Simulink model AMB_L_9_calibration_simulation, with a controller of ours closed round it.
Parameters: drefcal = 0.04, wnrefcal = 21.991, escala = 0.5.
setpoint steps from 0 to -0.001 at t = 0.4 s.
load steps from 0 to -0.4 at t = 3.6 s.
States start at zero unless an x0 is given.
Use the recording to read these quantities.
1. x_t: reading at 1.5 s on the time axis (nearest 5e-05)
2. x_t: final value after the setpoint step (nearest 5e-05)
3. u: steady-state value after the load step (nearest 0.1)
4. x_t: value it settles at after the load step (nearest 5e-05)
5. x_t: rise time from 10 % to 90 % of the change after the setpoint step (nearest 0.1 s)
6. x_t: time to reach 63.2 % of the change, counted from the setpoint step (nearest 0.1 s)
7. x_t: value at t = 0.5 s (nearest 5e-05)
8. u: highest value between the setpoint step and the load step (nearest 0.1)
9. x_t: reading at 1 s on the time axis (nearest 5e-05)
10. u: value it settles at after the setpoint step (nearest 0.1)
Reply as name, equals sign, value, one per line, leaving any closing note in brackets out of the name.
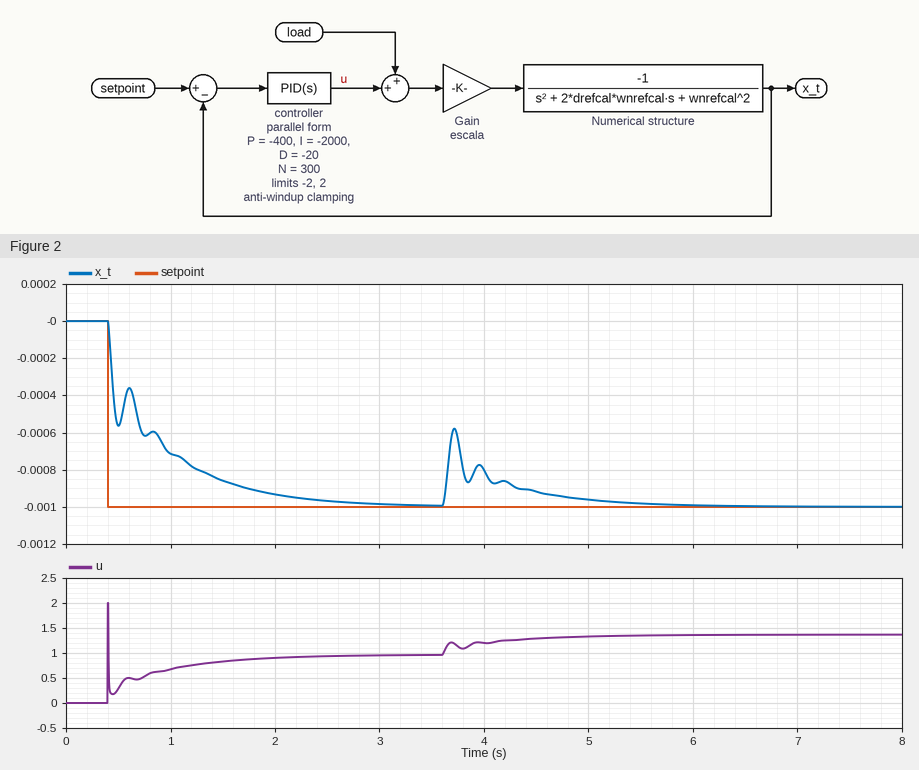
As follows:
x_t: reading at 1.5 s on the time axis = -0.00085
x_t: final value after the setpoint step = -0.00100
u: steady-state value after the load step = 1.4
x_t: value it settles at after the load step = -0.00100
x_t: rise time from 10 % to 90 % of the change after the setpoint step = 1.3 s
x_t: time to reach 63.2 % of the change, counted from the setpoint step = 0.5 s
x_t: value at t = 0.5 s = -0.00055
u: highest value between the setpoint step and the load step = 2.0
x_t: reading at 1 s on the time axis = -0.00070
u: value it settles at after the setpoint step = 1.0
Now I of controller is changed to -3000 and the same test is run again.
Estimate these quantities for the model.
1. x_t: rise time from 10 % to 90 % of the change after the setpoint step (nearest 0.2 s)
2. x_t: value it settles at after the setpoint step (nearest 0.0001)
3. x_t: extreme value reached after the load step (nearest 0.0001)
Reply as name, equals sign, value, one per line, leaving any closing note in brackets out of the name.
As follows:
x_t: rise time from 10 % to 90 % of the change after the setpoint step = 0.8 s
x_t: value it settles at after the setpoint step = -0.0010
x_t: extreme value reached after the load step = -0.0006
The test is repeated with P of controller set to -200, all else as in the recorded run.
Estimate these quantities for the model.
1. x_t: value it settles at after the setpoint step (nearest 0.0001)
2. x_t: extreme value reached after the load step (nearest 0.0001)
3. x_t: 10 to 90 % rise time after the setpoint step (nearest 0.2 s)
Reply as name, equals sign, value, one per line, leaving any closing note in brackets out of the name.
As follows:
x_t: value it settles at after the setpoint step = -0.0010
x_t: extreme value reached after the load step = -0.0005
x_t: 10 to 90 % rise time after the setpoint step = 1.2 s
